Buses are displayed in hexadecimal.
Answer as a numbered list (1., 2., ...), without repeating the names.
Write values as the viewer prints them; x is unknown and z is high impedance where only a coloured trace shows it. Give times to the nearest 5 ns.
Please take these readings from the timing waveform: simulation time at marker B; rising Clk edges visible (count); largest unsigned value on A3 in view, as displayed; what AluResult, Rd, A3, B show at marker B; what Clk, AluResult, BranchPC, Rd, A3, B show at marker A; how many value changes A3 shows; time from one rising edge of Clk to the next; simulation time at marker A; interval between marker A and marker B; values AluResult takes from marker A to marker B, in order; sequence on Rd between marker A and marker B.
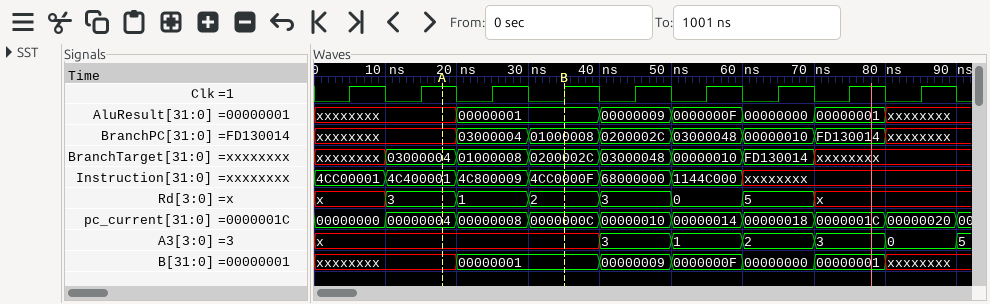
1. 35 ns
2. 9
3. 5
4. AluResult=00000001, Rd=2, A3=x, B=00000001
5. Clk=1, AluResult=xxxxxxxx, BranchPC=xxxxxxxx, Rd=3, A3=x, B=xxxxxxxx
6. 6
7. 10 ns
8. 20 ns
9. 15 ns
10. xxxxxxxx, 00000001
11. 3, 1, 2
